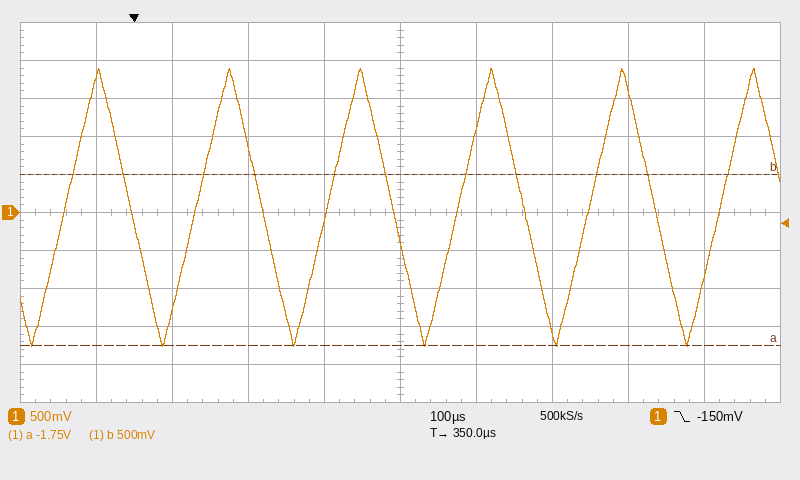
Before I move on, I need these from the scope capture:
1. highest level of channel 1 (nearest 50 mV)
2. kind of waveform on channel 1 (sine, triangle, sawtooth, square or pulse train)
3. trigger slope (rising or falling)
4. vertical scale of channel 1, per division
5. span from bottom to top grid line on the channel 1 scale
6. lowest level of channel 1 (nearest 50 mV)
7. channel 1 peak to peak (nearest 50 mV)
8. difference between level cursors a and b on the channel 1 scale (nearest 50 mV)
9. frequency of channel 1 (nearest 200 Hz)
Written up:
1.90 V
triangle
falling
500 mV
5 V
-1.75 V
3.65 V
2.25 V
5.8 kHz
